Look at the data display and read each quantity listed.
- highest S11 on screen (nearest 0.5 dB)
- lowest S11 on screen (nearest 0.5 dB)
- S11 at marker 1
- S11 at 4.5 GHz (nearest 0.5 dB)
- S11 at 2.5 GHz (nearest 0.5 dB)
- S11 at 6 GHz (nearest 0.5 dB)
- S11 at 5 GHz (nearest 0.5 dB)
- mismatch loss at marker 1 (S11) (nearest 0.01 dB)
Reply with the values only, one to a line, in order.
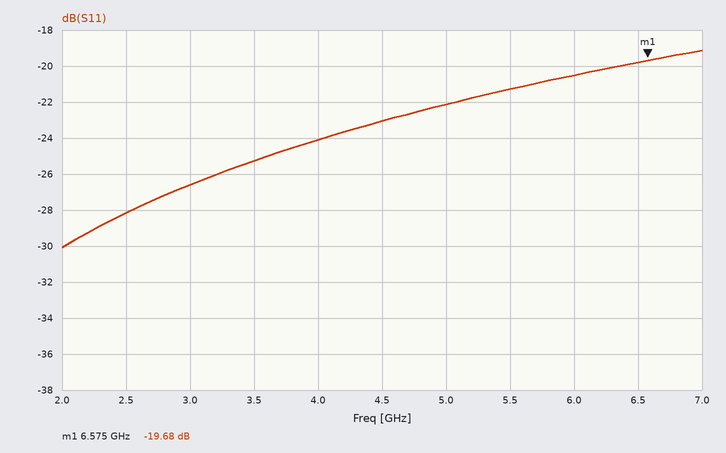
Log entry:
-19.0 dB
-30.0 dB
-19.68 dB
-23.0 dB
-28.0 dB
-20.5 dB
-22.0 dB
0.05 dB
